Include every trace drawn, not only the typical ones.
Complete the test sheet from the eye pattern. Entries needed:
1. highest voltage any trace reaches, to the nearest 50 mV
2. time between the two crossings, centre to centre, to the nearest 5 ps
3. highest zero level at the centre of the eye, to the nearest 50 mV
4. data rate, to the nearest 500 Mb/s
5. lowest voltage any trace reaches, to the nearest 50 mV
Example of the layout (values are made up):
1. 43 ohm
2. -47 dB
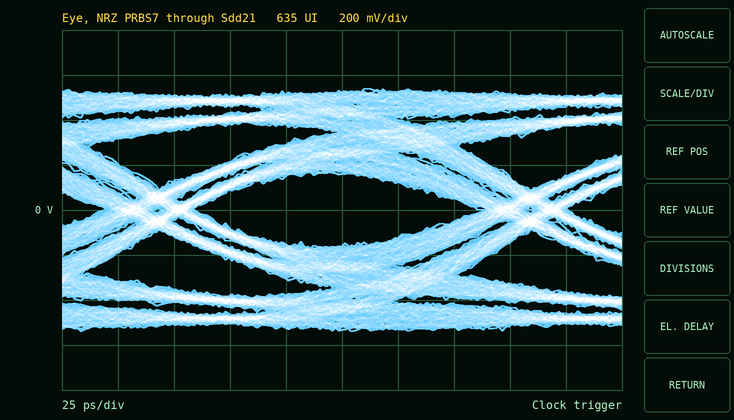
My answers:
1. 550 mV
2. 165 ps
3. -150 mV
4. 6.0 Gb/s
5. -550 mV
